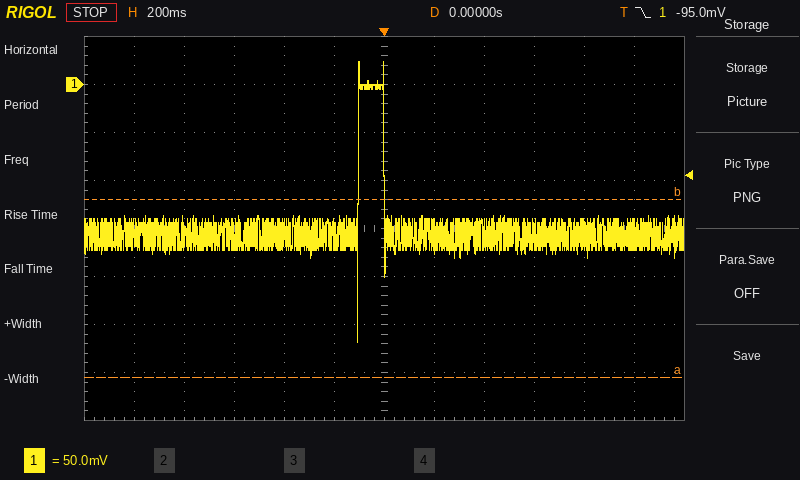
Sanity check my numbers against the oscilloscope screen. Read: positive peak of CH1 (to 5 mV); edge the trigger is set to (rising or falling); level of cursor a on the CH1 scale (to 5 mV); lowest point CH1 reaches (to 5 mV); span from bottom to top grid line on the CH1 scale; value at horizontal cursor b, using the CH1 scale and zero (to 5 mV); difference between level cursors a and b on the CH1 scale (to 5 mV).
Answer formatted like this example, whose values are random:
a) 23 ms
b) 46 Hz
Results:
a) 25 mV
b) falling
c) -305 mV
d) -270 mV
e) 400 mV
f) -120 mV
g) 185 mV
